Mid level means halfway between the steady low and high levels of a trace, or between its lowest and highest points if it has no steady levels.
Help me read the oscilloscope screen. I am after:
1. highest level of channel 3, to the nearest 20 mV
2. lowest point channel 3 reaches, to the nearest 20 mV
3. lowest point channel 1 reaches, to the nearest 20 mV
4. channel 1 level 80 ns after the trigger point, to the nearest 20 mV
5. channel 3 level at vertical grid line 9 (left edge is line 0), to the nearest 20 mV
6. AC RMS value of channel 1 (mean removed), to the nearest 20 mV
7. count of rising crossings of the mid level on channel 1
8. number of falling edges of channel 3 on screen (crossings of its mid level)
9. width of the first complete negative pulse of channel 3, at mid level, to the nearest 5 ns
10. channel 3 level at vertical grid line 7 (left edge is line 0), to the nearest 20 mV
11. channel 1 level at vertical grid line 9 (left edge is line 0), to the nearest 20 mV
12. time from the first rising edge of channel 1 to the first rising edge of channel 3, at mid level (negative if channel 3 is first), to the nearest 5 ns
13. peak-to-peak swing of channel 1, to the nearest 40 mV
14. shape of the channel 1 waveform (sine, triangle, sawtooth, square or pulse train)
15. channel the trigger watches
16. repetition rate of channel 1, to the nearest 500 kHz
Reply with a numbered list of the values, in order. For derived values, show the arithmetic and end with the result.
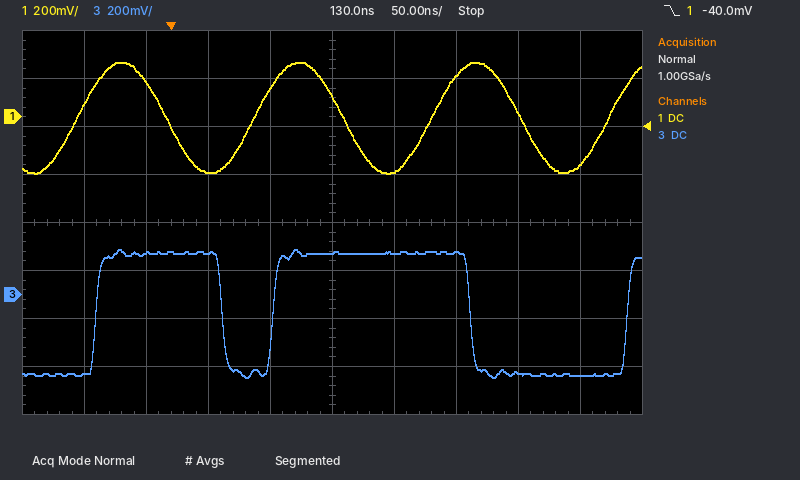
1. 180 mV
2. -340 mV
3. -240 mV
4. 120 mV
5. -340 mV
6. 480 mV / (2√2) ≈ 170 mV, so 160 mV to the nearest 20 mV
7. 4
8. 2
9. 40 ns
10. 180 mV
11. -200 mV
12. +15 ns
13. 480 mV
14. sine
15. channel 1
16. 7.0 MHz
